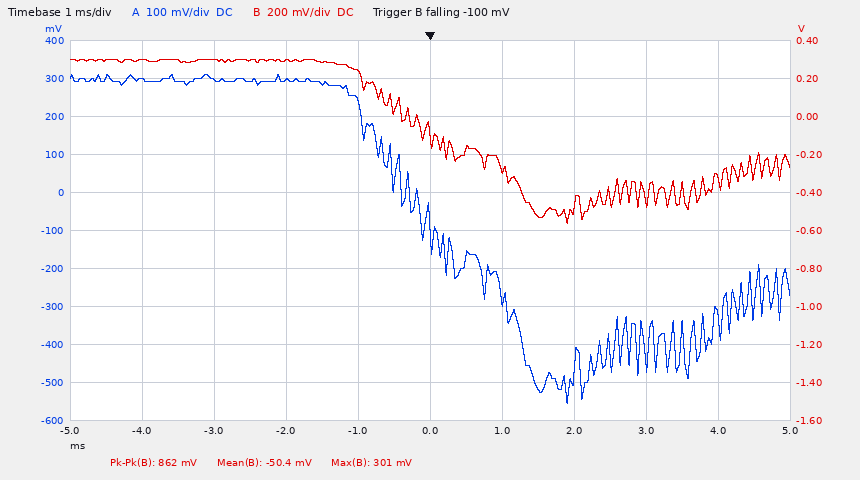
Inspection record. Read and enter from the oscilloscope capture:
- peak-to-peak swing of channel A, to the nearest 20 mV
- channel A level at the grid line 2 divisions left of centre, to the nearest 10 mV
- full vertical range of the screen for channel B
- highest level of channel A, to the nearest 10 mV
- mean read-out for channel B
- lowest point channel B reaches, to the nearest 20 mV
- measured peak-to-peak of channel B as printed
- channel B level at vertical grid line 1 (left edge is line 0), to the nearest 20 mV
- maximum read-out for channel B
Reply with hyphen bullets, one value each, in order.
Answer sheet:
- 860 mV
- 300 mV
- 2 V
- 310 mV
- -50.4 mV
- -560 mV
- 862 mV
- 300 mV
- 301 mV
